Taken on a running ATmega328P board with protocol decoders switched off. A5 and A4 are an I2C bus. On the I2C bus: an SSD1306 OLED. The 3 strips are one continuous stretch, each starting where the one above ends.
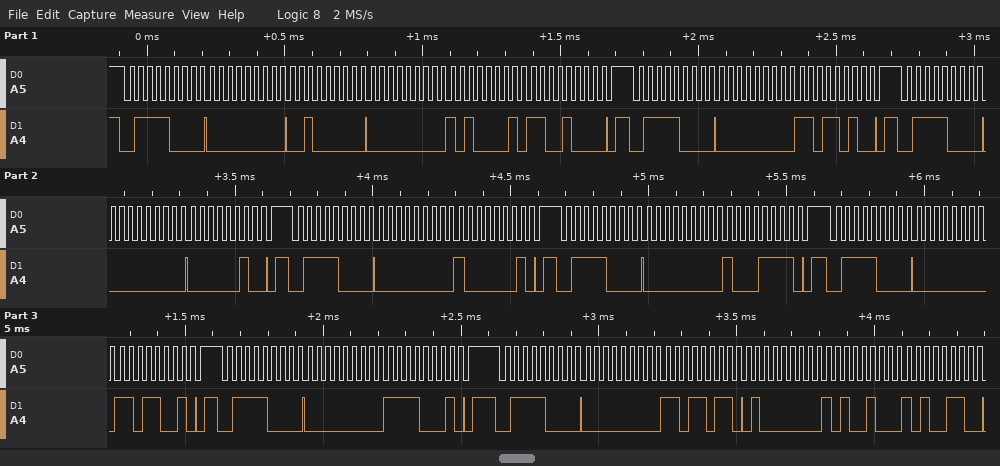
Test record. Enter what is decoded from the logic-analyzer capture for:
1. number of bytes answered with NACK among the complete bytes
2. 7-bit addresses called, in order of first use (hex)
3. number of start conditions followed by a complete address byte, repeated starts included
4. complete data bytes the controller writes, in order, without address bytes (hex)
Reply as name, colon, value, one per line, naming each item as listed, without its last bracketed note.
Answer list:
number of bytes answered with NACK among the complete bytes: 0
7-bit addresses called, in order of first use: 0x3C
number of start conditions followed by a complete address byte, repeated starts included: 8
complete data bytes the controller writes, in order, without address bytes: 00 20 00 A1 C8 00 DA 00 02 00 81 00 8F 00 D9 00 F1 00 DB 40 A4 A6
